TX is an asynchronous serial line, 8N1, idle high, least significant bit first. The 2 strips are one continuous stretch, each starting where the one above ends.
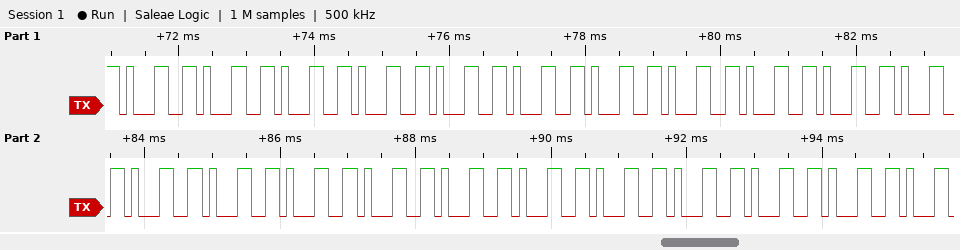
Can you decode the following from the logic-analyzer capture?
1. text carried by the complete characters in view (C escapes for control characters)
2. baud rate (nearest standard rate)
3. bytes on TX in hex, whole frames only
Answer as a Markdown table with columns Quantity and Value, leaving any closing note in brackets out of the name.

| Quantity | Value |
|---|---|
| text carried by the complete characters in view | "111111111111111111111" |
| baud rate | 9600 baud |
| bytes on TX in hex, whole frames only | 31 31 31 31 31 31 31 31 31 31 31 31 31 31 31 31 31 31 31 31 31 |
